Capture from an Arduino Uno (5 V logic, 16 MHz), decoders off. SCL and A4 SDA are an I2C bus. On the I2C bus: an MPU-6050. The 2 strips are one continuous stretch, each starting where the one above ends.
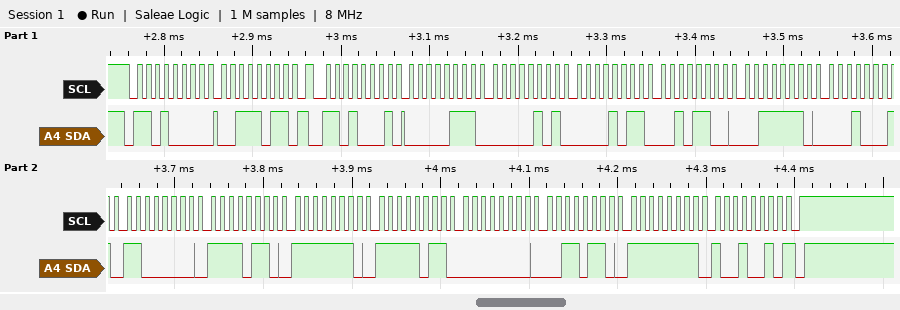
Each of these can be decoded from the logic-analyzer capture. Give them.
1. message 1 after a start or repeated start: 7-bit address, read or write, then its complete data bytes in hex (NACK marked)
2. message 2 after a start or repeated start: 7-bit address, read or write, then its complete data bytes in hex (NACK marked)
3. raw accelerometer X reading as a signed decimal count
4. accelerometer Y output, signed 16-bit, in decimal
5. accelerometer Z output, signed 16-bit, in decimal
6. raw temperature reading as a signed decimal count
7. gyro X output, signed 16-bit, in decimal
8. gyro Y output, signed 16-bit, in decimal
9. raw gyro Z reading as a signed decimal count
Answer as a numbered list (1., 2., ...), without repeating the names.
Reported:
1. 0x68 write: 3B
2. 0x68 read: 07 05 0B 2C 3E 11 C0 F6 FE FB 00 36 FF 92 NACK
3. 1797
4. 2860
5. 15889
6. -16138
7. -261
8. 54
9. -110
